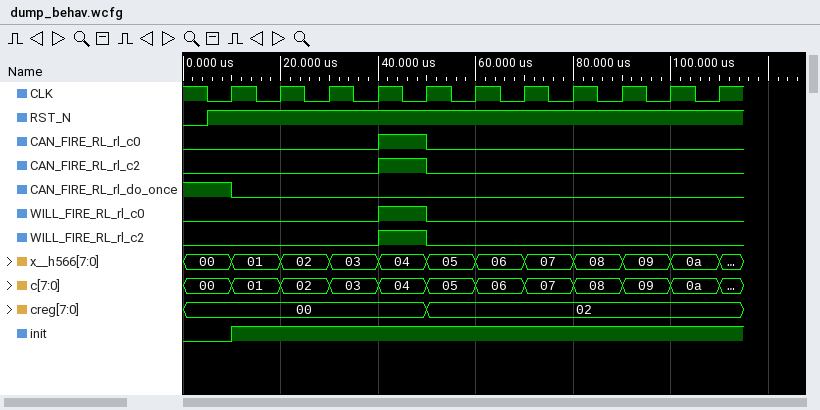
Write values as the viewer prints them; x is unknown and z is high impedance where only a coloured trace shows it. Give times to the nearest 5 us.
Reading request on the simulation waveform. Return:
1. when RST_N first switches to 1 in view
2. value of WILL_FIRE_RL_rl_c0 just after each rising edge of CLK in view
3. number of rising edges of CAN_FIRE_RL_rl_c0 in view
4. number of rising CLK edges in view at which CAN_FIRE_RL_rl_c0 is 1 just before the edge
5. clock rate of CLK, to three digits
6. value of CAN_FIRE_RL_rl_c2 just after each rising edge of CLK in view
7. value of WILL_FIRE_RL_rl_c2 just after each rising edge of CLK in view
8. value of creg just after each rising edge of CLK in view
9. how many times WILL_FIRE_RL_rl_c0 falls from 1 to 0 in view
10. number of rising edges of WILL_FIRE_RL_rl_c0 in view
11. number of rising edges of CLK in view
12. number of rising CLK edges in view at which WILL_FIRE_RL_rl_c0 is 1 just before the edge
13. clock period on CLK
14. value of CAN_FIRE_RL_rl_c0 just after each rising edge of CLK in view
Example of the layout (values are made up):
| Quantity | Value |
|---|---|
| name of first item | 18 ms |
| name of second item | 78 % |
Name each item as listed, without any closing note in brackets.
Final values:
| Quantity | Value |
|---|---|
| when RST_N first switches to 1 in view | 5 us |
| value of WILL_FIRE_RL_rl_c0 just after each rising edge of CLK in view | 0 0 0 1 0 0 0 0 0 0 0 |
| number of rising edges of CAN_FIRE_RL_rl_c0 in view | 1 |
| number of rising CLK edges in view at which CAN_FIRE_RL_rl_c0 is 1 just before the edge | 1 |
| clock rate of CLK, to three digits | 100 kHz |
| value of CAN_FIRE_RL_rl_c2 just after each rising edge of CLK in view | 0 0 0 1 0 0 0 0 0 0 0 |
| value of WILL_FIRE_RL_rl_c2 just after each rising edge of CLK in view | 0 0 0 1 0 0 0 0 0 0 0 |
| value of creg just after each rising edge of CLK in view | 00, 00, 00, 00, 02, 02, 02, 02, 02, 02, 02 |
| how many times WILL_FIRE_RL_rl_c0 falls from 1 to 0 in view | 1 |
| number of rising edges of WILL_FIRE_RL_rl_c0 in view | 1 |
| number of rising edges of CLK in view | 11 |
| number of rising CLK edges in view at which WILL_FIRE_RL_rl_c0 is 1 just before the edge | 1 |
| clock period on CLK | 10 us |
| value of CAN_FIRE_RL_rl_c0 just after each rising edge of CLK in view | 0 0 0 1 0 0 0 0 0 0 0 |
